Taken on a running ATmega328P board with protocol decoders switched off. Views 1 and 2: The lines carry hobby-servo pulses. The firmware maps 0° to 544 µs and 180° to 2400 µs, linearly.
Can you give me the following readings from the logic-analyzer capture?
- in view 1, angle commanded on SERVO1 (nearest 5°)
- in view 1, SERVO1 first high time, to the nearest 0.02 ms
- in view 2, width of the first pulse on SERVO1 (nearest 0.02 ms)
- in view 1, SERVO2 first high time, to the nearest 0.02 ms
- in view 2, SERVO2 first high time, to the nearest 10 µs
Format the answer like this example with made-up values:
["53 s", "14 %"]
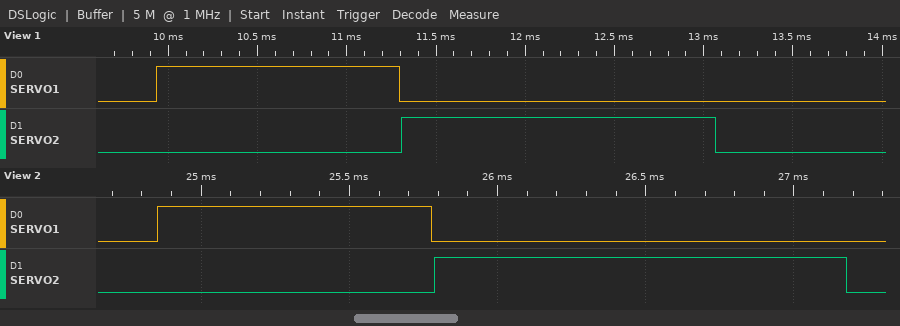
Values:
["80°", "1.36 ms", "0.92 ms", "1.76 ms", "1390 µs"]
